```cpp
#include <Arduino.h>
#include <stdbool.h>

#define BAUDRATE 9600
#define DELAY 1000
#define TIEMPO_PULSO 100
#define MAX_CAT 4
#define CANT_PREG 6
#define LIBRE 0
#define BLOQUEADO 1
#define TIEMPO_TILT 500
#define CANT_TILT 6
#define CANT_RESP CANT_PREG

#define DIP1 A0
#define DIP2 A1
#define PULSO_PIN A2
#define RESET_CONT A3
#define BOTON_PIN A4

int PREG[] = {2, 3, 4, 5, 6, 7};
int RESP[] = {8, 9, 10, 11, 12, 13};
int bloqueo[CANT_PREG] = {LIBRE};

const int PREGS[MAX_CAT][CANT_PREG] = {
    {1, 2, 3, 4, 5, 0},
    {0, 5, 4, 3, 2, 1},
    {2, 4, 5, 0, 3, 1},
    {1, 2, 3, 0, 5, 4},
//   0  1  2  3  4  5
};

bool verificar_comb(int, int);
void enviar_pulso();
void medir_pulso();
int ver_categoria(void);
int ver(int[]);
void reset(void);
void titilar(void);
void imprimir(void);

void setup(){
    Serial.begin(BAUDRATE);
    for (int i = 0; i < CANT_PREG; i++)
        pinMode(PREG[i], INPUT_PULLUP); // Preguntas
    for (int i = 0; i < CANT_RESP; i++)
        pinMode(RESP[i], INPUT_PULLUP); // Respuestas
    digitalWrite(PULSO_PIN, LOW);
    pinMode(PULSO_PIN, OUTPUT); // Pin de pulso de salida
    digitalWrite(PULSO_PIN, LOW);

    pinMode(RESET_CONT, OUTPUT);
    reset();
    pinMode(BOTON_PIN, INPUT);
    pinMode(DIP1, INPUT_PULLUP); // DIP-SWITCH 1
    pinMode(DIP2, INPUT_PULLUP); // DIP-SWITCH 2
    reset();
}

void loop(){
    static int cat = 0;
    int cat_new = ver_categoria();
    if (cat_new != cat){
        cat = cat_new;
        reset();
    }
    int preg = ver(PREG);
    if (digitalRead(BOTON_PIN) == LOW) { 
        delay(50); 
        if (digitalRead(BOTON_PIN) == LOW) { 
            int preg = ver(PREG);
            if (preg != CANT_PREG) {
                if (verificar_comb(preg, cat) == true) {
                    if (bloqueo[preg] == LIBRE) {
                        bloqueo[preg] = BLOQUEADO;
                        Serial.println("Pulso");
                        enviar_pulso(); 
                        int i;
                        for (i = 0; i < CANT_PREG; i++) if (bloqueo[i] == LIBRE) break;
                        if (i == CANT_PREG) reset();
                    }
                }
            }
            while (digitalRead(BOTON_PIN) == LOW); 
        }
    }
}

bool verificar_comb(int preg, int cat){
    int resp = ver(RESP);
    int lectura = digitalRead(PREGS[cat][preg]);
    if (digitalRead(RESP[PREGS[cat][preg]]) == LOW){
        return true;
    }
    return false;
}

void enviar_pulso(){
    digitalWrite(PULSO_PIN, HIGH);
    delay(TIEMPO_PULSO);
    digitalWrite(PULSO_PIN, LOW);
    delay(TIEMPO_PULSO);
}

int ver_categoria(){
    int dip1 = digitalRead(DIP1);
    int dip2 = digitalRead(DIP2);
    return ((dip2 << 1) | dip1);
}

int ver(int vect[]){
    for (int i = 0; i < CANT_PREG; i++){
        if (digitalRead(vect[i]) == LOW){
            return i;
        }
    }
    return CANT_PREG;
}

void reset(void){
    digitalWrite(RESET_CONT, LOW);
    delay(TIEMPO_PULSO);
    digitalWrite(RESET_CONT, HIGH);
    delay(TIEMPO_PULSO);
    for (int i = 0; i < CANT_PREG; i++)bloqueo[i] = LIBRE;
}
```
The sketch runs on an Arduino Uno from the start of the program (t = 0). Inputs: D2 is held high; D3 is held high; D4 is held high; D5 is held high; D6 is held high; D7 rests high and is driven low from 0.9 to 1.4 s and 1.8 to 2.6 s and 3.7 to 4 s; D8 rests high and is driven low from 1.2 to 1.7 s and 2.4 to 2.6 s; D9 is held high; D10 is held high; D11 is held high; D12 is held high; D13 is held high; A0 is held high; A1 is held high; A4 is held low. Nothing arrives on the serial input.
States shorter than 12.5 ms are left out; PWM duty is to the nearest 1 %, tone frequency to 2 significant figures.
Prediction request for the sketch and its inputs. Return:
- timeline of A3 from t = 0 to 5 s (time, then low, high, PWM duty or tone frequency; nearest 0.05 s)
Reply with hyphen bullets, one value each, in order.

- 0 s low; 0.1 s high; 0.2 s low; 0.3 s high; 0.4 s low; 0.5 s high
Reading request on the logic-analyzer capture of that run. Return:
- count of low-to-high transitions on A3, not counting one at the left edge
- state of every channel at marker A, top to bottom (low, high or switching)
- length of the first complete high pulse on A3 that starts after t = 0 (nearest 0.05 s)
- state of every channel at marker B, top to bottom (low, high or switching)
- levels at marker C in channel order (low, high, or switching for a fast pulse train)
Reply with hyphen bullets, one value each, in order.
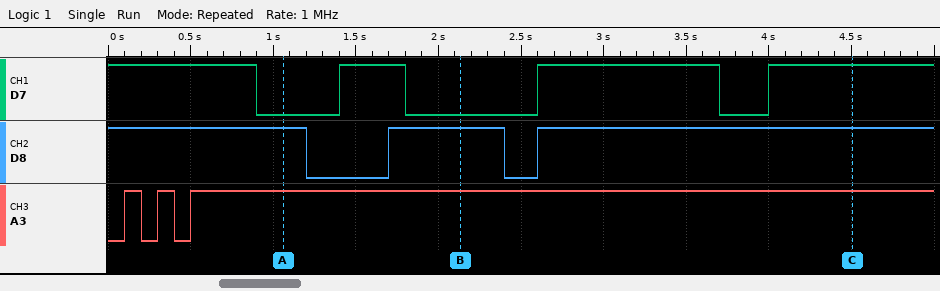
- 3
- D7 low, D8 high, A3 high
- 0.10 s
- D7 low, D8 high, A3 high
- D7 high, D8 high, A3 high
